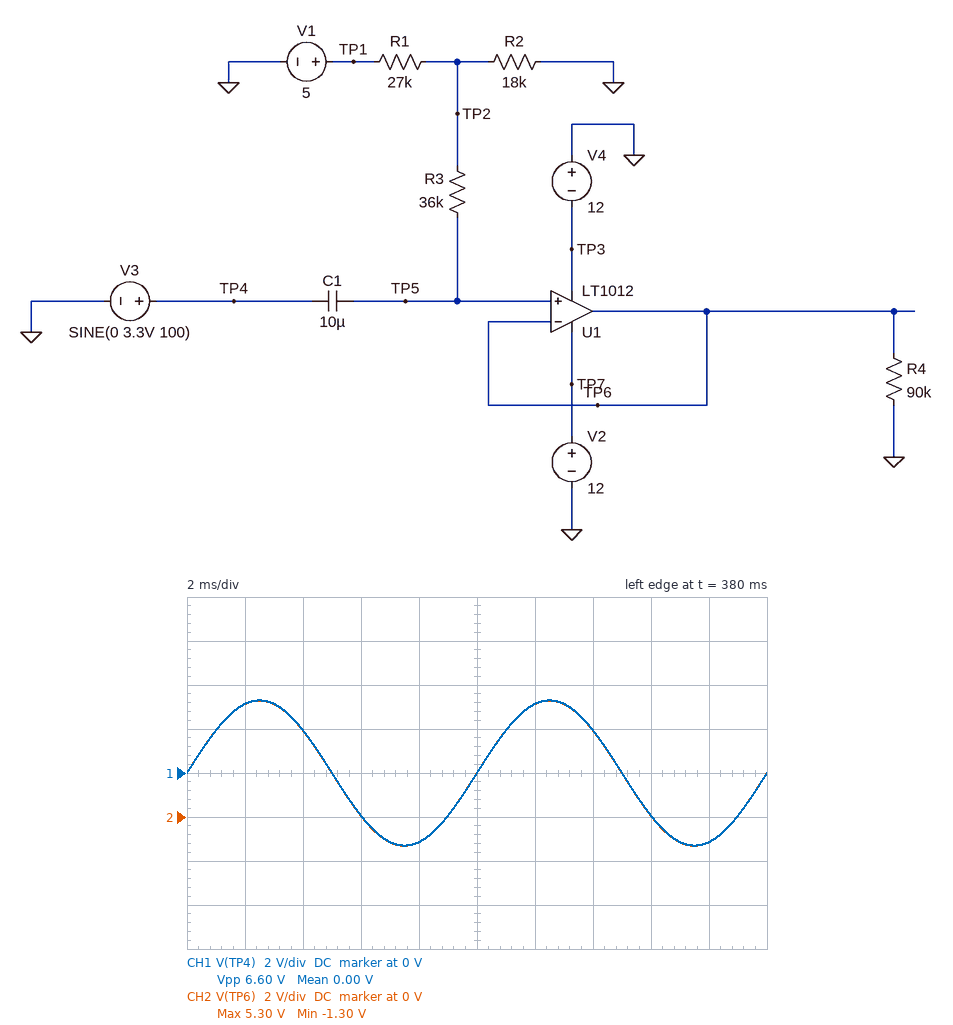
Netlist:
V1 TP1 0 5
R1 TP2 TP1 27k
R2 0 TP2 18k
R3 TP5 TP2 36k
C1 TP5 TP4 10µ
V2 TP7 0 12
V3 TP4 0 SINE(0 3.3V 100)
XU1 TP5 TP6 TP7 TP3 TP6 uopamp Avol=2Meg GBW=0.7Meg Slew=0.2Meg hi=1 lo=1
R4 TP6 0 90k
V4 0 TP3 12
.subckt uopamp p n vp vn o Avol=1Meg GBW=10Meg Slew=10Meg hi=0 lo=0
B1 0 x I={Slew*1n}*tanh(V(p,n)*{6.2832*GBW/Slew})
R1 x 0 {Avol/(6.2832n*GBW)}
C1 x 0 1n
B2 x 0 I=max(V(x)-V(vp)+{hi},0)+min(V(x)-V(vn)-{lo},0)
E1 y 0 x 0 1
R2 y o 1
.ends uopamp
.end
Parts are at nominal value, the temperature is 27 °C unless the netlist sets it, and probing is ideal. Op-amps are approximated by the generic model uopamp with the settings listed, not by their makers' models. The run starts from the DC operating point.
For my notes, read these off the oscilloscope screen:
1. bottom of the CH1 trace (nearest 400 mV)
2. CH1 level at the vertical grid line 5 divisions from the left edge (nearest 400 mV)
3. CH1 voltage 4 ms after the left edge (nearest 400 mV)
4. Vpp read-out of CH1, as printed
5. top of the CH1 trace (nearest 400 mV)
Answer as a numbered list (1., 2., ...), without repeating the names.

1. -3.2 V
2. 0 V
3. 2.0 V
4. 6.60 V
5. 3.2 V
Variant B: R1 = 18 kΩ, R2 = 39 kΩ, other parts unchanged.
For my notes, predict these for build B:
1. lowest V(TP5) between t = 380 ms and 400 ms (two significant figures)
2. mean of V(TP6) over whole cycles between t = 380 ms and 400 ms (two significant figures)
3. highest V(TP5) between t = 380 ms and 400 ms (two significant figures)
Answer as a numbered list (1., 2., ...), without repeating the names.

1. 120 mV
2. 3.4 V
3. 6.7 V
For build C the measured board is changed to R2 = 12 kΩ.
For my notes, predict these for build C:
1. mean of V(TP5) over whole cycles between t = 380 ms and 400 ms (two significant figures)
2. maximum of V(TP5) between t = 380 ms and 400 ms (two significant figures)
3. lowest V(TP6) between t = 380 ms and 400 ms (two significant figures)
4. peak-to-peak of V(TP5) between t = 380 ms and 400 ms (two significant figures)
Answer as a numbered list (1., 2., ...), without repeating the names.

1. 1.5 V
2. 4.8 V
3. -1.8 V
4. 6.6 V
